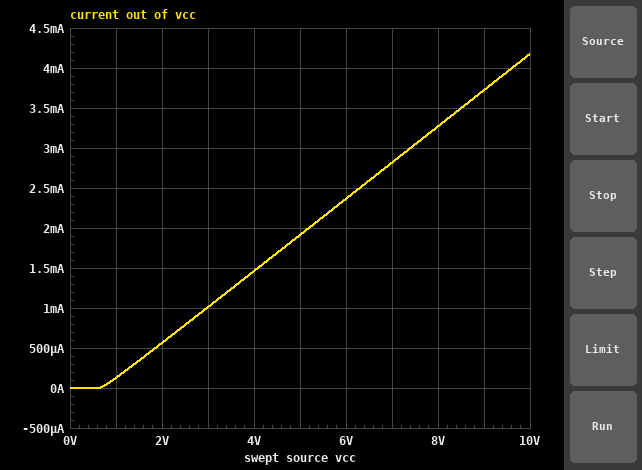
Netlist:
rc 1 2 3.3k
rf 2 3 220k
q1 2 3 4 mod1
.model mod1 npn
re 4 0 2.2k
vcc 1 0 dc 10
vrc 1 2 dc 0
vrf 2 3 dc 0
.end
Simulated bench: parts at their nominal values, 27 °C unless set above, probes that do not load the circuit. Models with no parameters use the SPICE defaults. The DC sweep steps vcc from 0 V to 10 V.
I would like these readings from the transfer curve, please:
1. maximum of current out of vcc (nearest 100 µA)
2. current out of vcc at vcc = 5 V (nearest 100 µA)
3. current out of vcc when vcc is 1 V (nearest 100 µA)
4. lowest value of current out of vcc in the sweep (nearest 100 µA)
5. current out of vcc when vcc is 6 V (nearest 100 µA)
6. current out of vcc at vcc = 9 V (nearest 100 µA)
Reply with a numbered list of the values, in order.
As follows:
1. 4.2 mA
2. 1.9 mA
3. 100 µA
4. 0 A
5. 2.4 mA
6. 3.7 mA
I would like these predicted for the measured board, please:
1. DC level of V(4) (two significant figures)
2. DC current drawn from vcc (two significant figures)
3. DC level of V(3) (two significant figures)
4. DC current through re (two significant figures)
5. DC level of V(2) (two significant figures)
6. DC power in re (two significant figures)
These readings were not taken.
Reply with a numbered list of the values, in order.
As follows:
1. 9.2 V
2. 4.2 mA
3. 10 V
4. 4.2 mA
5. 10 V
6. 38 mW
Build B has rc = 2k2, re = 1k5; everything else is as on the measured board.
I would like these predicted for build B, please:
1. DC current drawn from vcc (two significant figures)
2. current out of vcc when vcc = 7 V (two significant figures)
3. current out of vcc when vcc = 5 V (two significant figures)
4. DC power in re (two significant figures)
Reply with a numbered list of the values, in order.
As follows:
1. 6.1 mA
2. 4.1 mA
3. 2.8 mA
4. 56 mW
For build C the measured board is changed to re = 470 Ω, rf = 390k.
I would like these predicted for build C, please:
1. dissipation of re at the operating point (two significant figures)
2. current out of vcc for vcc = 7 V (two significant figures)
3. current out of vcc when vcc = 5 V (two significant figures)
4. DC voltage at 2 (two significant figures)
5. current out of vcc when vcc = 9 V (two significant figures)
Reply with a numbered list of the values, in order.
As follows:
1. 180 mW
2. 13 mA
3. 8.9 mA
4. 10 V
5. 17 mA
